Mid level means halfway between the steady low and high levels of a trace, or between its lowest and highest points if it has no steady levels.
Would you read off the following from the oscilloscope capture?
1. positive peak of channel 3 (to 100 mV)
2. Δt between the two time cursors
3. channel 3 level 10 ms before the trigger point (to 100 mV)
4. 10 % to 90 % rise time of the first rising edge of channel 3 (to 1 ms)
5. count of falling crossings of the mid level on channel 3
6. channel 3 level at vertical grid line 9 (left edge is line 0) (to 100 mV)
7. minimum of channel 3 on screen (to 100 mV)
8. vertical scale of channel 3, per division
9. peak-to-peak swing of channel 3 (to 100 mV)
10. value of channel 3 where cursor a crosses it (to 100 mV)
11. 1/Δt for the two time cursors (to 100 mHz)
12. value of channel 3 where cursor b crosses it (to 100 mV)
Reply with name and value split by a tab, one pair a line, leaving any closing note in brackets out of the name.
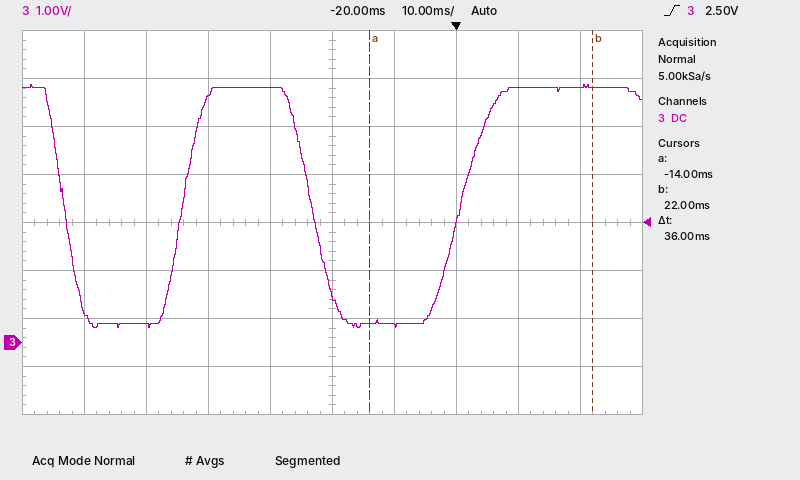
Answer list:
positive peak of channel 3	5.4 V
Δt between the two time cursors	36 ms
channel 3 level 10 ms before the trigger point	400 mV
10 % to 90 % rise time of the first rising edge of channel 3	6 ms
count of falling crossings of the mid level on channel 3	2
channel 3 level at vertical grid line 9 (left edge is line 0)	5.3 V
minimum of channel 3 on screen	300 mV
vertical scale of channel 3, per division	1 V
peak-to-peak swing of channel 3	5.1 V
value of channel 3 where cursor a crosses it	400 mV
1/Δt for the two time cursors	27.8 Hz
value of channel 3 where cursor b crosses it	5.3 V
